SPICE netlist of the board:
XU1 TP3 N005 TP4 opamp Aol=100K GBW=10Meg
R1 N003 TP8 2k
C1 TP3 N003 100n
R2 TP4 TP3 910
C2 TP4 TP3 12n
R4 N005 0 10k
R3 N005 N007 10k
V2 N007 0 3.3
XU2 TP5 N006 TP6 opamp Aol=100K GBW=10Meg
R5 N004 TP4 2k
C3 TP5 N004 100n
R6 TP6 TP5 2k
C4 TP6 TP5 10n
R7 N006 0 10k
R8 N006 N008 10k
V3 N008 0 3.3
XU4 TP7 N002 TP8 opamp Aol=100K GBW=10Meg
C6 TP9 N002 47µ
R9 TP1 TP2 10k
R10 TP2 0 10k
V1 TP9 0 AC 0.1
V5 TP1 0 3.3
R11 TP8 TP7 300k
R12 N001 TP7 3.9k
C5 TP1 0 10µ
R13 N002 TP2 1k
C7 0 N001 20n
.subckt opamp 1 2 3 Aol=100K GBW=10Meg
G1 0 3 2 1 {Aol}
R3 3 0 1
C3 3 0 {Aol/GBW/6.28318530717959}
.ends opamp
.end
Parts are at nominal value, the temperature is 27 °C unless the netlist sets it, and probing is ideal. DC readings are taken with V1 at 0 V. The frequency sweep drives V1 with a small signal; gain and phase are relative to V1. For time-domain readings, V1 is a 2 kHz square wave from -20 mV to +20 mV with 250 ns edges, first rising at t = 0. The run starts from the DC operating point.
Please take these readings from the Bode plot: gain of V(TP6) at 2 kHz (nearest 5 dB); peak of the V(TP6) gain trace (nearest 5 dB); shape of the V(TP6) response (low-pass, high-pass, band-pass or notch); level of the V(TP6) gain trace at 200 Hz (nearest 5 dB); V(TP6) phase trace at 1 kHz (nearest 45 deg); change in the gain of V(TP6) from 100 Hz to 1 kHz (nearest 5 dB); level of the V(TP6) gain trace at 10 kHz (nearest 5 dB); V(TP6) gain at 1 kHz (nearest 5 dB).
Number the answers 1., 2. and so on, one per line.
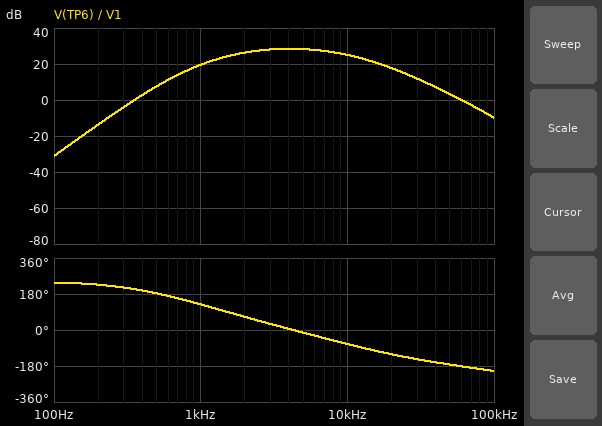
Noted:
1. 25 dB
2. 30 dB
3. band-pass
4. -15 dB
5. 135 deg
6. 50 dB
7. 25 dB
8. 20 dB
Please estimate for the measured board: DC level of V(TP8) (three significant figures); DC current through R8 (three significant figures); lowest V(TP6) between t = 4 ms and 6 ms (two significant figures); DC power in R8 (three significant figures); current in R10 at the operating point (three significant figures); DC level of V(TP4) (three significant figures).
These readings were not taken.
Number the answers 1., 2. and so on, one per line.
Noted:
1. 1.65 V
2. 165 µA
3. 810 mV
4. 272 µW
5. 165 µA
6. 1.65 V
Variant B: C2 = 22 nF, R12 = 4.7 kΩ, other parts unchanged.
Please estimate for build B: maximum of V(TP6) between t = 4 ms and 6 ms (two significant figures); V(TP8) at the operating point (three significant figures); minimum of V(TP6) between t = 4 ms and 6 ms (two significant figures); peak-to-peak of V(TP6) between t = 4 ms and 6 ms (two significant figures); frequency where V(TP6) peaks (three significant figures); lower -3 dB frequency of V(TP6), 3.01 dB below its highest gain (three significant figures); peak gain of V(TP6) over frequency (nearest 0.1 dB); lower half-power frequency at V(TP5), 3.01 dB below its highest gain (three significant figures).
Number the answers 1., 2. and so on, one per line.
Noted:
1. 2.3 V
2. 1.65 V
3. 980 mV
4. 1.3 V
5. 3.39 kHz
6. 1.53 kHz
7. 26.6 dB
8. 3.83 kHz
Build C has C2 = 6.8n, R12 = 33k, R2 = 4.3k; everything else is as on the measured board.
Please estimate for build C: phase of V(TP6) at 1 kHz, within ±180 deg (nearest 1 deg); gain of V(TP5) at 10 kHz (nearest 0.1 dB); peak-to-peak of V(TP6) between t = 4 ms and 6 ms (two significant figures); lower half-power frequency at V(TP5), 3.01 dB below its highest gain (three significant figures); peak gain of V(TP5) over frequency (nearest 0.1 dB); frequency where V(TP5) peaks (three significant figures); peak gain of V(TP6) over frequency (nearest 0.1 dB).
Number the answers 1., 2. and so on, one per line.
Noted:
1. 72 deg
2. -43.9 dB
3. 990 mV
4. 2.93 kHz
5. -43.2 dB
6. 6.77 kHz
7. 24.6 dB
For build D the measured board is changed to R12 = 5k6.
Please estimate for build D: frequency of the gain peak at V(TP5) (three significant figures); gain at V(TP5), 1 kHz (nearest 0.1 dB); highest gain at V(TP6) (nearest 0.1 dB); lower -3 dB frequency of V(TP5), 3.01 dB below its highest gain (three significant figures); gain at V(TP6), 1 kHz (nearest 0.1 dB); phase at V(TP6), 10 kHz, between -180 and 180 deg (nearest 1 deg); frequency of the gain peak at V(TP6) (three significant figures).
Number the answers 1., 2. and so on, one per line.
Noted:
1. 11.0 kHz
2. -61.2 dB
3. 25.8 dB
4. 4.70 kHz
5. 18.8 dB
6. -72 deg
7. 3.61 kHz
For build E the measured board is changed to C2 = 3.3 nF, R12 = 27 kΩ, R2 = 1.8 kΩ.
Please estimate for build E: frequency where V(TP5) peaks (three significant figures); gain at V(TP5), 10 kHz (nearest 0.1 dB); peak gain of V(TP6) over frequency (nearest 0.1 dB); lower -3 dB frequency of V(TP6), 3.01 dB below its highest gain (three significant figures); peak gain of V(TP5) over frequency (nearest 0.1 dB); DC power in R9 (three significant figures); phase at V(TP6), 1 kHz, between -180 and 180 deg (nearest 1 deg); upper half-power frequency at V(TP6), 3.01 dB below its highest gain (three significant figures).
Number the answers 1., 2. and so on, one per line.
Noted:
1. 14.7 kHz
2. -44.0 dB
3. 19.5 dB
4. 1.06 kHz
5. -43.5 dB
6. 272 µW
7. 83 deg
8. 9.25 kHz
